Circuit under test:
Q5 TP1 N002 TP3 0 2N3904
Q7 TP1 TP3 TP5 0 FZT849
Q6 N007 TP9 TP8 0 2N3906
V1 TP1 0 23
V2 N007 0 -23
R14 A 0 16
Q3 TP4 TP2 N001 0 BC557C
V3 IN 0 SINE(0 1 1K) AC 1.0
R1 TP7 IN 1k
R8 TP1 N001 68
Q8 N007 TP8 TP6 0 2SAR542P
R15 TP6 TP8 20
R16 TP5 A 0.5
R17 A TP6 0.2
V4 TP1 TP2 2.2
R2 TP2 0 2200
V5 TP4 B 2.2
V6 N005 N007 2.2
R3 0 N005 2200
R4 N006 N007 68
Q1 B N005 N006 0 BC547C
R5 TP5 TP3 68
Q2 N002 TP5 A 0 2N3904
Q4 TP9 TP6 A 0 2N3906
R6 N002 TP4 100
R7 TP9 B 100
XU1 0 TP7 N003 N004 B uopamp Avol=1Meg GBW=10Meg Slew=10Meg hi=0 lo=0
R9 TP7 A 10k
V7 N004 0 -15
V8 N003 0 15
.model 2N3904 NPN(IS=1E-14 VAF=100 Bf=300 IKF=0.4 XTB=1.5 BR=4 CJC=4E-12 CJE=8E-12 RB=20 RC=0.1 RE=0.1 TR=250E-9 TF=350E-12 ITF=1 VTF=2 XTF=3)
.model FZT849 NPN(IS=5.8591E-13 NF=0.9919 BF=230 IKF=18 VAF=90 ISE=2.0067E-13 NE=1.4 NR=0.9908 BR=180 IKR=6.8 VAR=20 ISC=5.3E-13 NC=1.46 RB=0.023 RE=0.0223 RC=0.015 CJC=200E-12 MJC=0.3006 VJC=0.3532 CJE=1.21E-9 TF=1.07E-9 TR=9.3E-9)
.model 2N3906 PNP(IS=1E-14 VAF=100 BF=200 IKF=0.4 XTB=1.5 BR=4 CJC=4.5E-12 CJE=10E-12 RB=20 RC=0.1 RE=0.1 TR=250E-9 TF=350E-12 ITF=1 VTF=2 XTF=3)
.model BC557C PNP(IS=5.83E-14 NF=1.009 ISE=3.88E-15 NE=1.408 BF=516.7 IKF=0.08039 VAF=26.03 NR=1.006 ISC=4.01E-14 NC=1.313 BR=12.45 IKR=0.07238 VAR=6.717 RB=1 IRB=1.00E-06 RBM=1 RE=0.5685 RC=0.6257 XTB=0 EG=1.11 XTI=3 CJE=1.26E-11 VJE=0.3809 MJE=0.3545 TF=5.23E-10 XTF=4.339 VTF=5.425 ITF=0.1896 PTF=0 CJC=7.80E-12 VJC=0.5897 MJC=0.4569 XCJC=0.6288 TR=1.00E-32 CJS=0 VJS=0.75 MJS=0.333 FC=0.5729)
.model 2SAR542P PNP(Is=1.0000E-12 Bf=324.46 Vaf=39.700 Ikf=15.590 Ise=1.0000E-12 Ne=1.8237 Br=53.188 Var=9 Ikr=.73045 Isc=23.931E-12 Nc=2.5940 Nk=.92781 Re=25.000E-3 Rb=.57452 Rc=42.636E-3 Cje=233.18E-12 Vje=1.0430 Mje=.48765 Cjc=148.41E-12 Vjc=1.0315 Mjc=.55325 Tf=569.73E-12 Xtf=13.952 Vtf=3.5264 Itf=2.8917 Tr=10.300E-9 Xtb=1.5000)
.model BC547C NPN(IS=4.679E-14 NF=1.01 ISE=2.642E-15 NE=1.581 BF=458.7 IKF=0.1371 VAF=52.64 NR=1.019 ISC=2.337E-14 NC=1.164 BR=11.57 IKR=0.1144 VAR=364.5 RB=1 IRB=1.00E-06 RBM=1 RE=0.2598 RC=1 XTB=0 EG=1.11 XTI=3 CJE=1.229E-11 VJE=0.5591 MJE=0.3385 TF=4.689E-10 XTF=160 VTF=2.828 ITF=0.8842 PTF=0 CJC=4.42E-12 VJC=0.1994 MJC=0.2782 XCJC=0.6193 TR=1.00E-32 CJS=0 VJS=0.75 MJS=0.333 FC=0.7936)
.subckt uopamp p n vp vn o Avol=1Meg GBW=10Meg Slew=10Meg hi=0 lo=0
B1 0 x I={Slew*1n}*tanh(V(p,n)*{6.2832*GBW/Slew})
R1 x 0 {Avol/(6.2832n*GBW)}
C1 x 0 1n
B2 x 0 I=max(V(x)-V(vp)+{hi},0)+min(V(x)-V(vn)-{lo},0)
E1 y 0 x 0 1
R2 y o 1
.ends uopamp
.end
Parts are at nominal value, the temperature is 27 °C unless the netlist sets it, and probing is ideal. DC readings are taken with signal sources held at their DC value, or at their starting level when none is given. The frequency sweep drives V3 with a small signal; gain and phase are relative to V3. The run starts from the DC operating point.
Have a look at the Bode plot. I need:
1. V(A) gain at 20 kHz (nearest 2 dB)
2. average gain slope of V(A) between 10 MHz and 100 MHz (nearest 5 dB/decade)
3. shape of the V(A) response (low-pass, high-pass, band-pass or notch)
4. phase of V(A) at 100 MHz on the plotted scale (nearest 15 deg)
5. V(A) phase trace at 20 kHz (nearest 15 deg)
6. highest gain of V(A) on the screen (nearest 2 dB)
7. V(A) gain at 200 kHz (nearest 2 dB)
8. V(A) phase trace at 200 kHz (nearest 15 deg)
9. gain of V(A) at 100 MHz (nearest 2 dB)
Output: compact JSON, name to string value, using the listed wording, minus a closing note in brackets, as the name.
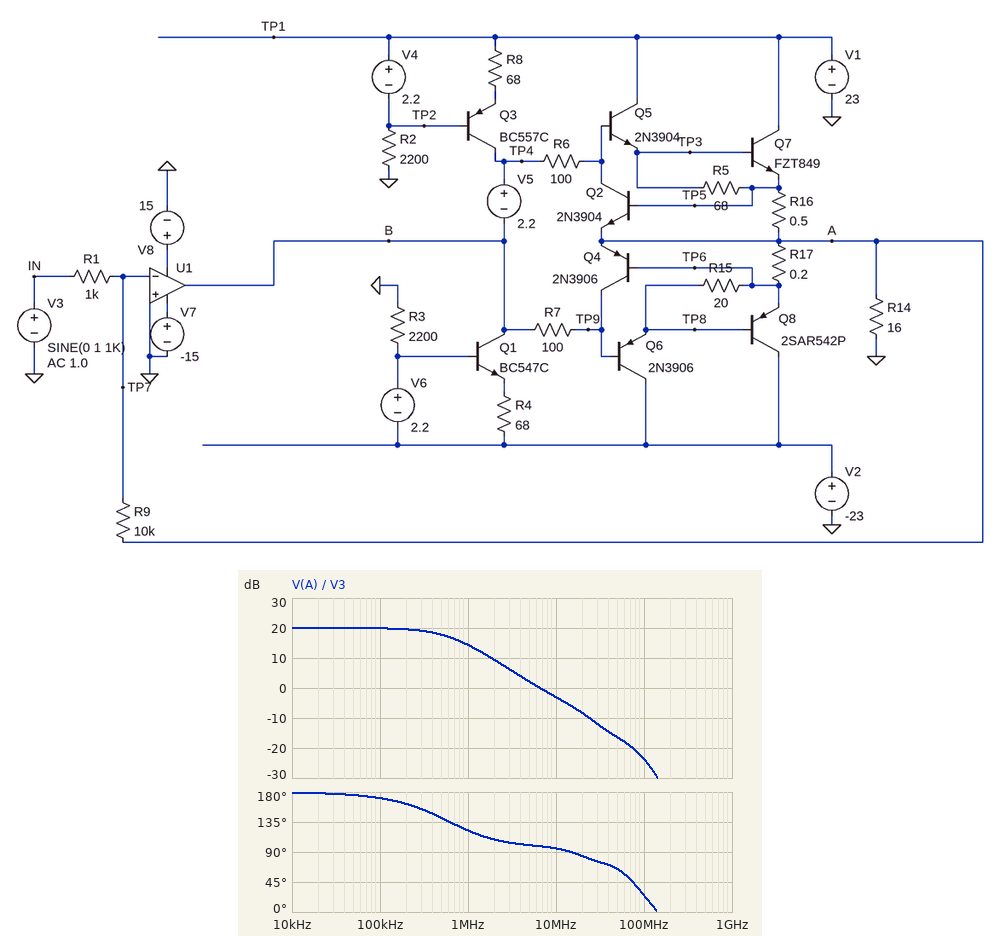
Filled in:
{"V(A) gain at 20 kHz": "20 dB", "average gain slope of V(A) between 10 MHz and 100 MHz": "-20 dB/decade", "shape of the V(A) response": "low-pass", "phase of V(A) at 100 MHz on the plotted scale": "30 deg", "V(A) phase trace at 20 kHz": "180 deg", "highest gain of V(A) on the screen": "20 dB", "V(A) gain at 200 kHz": "20 dB", "V(A) phase trace at 200 kHz": "165 deg", "gain of V(A) at 100 MHz": "-24 dB"}
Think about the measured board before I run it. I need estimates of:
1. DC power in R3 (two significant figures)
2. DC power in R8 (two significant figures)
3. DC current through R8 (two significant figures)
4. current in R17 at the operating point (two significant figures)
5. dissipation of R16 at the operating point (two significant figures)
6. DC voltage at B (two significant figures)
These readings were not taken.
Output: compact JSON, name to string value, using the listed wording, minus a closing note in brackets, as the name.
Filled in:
{"DC power in R3": "200 mW", "DC power in R8": "33 mW", "DC current through R8": "22 mA", "current in R17 at the operating point": "10 mA", "dissipation of R16 at the operating point": "54 µW", "DC voltage at B": "-930 mV"}
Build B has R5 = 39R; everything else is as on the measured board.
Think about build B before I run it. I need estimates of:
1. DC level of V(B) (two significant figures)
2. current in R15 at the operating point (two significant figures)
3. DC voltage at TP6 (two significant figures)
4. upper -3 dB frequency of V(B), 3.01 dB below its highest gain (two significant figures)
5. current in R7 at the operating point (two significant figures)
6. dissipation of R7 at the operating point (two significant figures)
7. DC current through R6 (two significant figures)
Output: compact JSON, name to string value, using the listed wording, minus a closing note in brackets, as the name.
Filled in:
{"DC level of V(B)": "-980 mV", "current in R15 at the operating point": "13 mA", "DC voltage at TP6": "-2.5 mV", "upper -3 dB frequency of V(B), 3.01 dB below its highest gain": "470 kHz", "current in R7 at the operating point": "53 µA", "dissipation of R7 at the operating point": "280 nW", "DC current through R6": "35 µA"}
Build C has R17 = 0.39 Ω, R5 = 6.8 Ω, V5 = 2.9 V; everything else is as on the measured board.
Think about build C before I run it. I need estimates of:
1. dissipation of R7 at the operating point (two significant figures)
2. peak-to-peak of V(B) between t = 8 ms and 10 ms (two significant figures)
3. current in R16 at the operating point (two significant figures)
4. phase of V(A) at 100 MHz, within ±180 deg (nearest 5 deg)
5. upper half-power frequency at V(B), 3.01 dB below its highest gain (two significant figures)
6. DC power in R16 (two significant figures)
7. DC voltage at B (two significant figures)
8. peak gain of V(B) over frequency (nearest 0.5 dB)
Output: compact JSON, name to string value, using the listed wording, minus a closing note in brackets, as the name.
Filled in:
{"dissipation of R7 at the operating point": "1.9 µW", "peak-to-peak of V(B) between t = 8 ms and 10 ms": "21 V", "current in R16 at the operating point": "99 mA", "phase of V(A) at 100 MHz, within ±180 deg": "10 deg", "upper half-power frequency at V(B), 3.01 dB below its highest gain": "880 kHz", "DC power in R16": "4.9 mW", "DC voltage at B": "-1.4 V", "peak gain of V(B) over frequency": "20.5 dB"}
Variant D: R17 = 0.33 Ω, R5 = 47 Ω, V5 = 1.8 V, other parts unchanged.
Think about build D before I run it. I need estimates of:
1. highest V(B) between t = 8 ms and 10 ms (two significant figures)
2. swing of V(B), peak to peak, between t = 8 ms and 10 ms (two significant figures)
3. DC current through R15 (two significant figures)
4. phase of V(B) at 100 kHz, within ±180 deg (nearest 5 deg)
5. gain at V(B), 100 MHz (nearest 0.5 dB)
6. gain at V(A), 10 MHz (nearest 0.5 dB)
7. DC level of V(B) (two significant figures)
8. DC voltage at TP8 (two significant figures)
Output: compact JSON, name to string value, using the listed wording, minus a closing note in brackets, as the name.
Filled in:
{"highest V(B) between t = 8 ms and 10 ms": "10 V", "swing of V(B), peak to peak, between t = 8 ms and 10 ms": "22 V", "DC current through R15": "5.9 mA", "phase of V(B) at 100 kHz, within ±180 deg": "165 deg", "gain at V(B), 100 MHz": "-21.0 dB", "gain at V(A), 10 MHz": "-4.0 dB", "DC level of V(B)": "-820 mV", "DC voltage at TP8": "-120 mV"}
